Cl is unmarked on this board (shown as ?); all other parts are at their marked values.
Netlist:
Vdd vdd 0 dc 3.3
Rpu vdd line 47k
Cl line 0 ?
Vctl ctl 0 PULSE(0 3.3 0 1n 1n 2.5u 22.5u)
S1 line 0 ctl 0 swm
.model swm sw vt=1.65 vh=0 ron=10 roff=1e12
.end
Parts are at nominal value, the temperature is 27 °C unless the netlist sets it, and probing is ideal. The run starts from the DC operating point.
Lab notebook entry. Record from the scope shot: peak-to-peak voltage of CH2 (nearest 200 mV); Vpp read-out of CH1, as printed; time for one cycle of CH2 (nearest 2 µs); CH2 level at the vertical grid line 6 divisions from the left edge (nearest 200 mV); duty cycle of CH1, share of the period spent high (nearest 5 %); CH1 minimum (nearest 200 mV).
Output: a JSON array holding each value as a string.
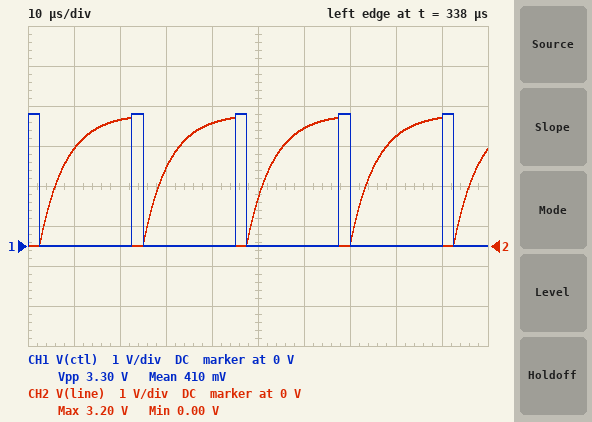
["3.2 V", "3.30 V", "22 µs", "3.0 V", "10 %", "0 V"]
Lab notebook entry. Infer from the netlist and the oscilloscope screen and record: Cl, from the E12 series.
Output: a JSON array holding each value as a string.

["120 pF"]
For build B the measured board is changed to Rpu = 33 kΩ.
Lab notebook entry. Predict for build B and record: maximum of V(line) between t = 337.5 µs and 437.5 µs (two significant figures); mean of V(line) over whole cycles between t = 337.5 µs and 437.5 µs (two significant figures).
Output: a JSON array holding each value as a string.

["3.3 V", "2.4 V"]
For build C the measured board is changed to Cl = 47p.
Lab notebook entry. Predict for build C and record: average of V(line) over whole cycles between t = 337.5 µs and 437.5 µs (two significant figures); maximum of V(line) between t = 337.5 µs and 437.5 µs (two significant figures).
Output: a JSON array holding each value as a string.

["2.6 V", "3.3 V"]
